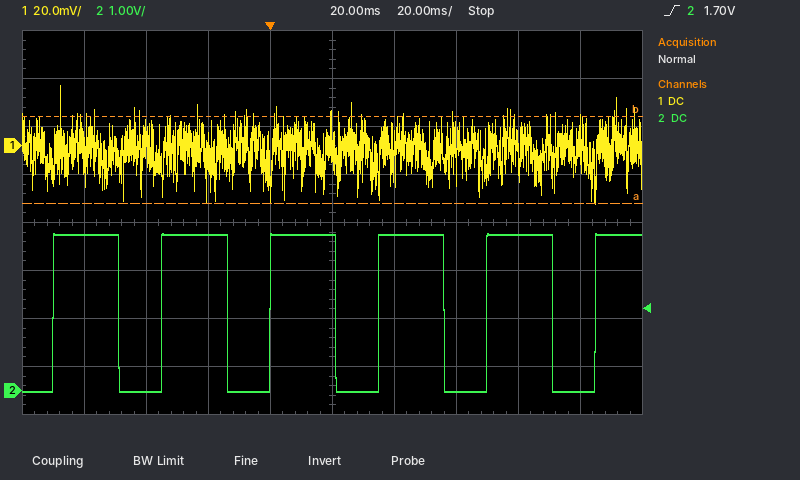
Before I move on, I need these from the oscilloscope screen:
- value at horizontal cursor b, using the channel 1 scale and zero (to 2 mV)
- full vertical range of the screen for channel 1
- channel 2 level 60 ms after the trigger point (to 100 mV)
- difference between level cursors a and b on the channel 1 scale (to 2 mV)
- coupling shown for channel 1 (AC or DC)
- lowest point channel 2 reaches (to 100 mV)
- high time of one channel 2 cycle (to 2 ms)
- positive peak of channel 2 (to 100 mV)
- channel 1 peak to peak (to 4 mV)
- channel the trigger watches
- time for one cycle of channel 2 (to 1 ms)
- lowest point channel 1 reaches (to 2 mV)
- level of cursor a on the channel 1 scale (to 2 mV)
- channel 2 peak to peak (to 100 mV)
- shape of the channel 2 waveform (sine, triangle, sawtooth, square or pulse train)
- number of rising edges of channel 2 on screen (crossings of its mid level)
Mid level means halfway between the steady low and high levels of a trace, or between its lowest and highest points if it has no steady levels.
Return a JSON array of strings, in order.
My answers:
["12 mV", "160 mV", "0.0 V", "36 mV", "DC", "0.0 V", "22 ms", "3.3 V", "48 mV", "channel 2", "35 ms", "-24 mV", "-24 mV", "3.3 V", "pulse train", "6"]
